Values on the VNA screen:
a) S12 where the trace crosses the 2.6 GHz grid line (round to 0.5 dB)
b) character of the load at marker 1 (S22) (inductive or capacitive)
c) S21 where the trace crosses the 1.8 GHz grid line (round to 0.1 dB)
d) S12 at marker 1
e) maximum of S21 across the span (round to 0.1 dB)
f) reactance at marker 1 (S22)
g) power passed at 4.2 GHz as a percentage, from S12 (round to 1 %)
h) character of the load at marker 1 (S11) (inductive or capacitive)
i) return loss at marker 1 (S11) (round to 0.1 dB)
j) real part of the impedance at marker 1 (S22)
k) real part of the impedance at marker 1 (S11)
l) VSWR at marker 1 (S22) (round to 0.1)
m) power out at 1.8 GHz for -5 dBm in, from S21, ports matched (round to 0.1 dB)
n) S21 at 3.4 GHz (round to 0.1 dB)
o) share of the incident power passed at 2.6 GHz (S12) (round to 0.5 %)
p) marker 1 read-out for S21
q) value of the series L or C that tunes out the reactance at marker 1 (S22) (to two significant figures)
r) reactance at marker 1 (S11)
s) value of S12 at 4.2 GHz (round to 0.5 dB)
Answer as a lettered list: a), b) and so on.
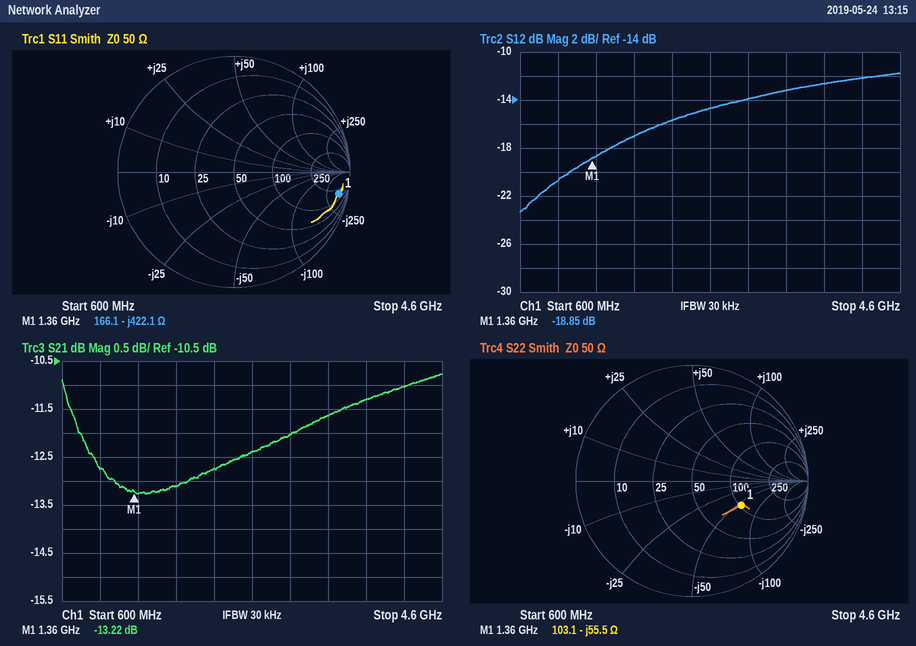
a) -14.5 dB
b) capacitive
c) -13.1 dB
d) -18.85 dB
e) -10.8 dB
f) -55.5 Ω
g) 6 %
h) capacitive
i) 0.7 dB
j) 103.1 Ω
k) 166.1 Ω
l) 2.8
m) -18.1 dBm
n) -11.6 dB
o) 3.5 %
p) -13.22 dB
q) 6.5 nH
r) -422.1 Ω
s) -12.0 dB
